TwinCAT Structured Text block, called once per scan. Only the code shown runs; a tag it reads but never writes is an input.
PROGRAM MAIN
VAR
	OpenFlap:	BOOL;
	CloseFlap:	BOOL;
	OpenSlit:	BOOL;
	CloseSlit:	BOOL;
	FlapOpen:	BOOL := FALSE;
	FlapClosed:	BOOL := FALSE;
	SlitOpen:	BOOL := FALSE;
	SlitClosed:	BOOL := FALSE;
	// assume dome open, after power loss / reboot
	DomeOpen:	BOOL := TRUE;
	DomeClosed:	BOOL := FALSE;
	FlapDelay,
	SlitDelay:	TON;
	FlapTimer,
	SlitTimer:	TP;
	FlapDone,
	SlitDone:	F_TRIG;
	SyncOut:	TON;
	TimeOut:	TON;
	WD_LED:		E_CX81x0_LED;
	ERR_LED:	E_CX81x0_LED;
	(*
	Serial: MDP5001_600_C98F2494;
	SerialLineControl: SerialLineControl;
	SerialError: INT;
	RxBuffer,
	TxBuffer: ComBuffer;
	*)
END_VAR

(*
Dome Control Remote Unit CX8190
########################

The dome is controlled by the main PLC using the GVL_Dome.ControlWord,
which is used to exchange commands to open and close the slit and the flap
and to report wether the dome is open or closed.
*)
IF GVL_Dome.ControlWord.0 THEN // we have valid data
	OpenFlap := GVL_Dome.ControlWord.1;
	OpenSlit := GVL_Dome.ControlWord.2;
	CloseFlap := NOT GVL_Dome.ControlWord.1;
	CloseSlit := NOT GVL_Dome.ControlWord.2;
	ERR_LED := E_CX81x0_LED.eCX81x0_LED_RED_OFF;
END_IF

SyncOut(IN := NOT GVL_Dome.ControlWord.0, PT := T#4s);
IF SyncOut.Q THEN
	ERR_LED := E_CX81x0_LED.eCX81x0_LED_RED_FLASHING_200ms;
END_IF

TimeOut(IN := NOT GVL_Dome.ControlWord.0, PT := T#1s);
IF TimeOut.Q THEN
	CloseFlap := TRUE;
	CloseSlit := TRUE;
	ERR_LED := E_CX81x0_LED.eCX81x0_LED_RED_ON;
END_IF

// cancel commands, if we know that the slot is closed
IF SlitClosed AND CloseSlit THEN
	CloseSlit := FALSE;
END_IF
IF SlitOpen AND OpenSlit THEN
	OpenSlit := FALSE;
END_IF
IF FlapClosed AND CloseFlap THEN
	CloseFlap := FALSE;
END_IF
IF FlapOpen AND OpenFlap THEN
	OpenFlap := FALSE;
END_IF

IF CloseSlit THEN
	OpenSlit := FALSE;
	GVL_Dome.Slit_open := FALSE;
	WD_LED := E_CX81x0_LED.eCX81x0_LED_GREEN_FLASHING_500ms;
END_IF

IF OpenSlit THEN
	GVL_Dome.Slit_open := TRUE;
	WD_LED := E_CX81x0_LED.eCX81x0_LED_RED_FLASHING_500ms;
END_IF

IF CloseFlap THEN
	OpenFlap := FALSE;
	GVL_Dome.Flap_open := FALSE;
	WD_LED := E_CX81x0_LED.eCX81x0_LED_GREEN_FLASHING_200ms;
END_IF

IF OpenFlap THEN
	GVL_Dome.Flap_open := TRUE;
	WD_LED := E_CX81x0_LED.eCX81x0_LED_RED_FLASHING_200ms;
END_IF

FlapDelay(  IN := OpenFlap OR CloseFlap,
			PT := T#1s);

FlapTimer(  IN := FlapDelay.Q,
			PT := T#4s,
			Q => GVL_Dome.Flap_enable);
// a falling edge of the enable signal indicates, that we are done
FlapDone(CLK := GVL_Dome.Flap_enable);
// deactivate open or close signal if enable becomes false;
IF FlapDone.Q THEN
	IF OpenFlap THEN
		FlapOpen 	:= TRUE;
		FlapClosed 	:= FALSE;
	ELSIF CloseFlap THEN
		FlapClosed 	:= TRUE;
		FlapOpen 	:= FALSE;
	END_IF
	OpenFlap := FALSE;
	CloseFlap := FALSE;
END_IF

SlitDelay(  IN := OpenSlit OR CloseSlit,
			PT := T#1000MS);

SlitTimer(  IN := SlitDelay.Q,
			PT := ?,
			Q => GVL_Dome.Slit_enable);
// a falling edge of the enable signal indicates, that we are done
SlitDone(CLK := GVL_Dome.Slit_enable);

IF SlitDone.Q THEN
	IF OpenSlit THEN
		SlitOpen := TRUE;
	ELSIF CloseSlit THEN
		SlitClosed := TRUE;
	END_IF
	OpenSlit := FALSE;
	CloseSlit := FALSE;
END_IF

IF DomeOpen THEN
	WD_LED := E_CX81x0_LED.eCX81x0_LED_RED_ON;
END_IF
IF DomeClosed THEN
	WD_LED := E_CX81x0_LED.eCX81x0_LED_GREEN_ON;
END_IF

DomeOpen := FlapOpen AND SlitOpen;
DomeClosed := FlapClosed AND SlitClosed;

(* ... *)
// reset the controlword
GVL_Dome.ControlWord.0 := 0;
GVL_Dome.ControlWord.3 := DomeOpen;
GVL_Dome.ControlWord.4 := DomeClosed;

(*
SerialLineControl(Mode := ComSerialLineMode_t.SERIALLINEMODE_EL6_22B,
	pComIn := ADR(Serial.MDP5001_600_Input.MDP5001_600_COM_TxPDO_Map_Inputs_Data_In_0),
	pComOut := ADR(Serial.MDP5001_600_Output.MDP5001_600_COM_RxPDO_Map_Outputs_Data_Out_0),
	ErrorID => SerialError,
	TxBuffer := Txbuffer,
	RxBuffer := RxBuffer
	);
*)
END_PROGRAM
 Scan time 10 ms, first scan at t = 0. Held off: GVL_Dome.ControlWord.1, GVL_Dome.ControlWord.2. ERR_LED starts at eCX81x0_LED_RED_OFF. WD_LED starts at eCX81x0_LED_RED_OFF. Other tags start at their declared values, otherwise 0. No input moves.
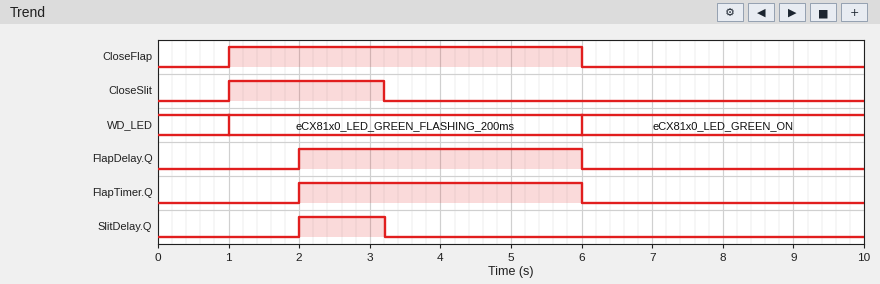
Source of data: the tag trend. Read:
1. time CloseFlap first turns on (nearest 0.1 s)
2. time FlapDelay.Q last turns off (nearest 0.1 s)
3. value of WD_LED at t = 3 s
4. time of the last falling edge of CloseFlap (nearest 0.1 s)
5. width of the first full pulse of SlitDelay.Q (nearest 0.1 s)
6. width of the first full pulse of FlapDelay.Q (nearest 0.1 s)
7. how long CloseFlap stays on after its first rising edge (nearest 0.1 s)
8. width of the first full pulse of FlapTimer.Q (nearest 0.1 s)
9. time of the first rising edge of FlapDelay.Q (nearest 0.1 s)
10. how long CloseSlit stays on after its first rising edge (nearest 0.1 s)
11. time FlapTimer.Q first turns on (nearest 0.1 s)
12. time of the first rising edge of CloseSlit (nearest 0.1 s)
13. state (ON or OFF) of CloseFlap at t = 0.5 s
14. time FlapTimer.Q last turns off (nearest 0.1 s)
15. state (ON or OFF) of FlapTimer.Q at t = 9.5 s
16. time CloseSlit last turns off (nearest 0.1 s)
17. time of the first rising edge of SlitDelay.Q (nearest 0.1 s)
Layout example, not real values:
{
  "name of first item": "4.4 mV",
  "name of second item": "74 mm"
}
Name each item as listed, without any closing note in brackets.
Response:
{
  "time CloseFlap first turns on": "1.0 s",
  "time FlapDelay.Q last turns off": "6.0 s",
  "value of WD_LED at t = 3 s": "eCX81x0_LED_GREEN_FLASHING_200ms",
  "time of the last falling edge of CloseFlap": "6.0 s",
  "width of the first full pulse of SlitDelay.Q": "1.2 s",
  "width of the first full pulse of FlapDelay.Q": "4.0 s",
  "how long CloseFlap stays on after its first rising edge": "5.0 s",
  "width of the first full pulse of FlapTimer.Q": "4.0 s",
  "time of the first rising edge of FlapDelay.Q": "2.0 s",
  "how long CloseSlit stays on after its first rising edge": "2.2 s",
  "time FlapTimer.Q first turns on": "2.0 s",
  "time of the first rising edge of CloseSlit": "1.0 s",
  "state (ON or OFF) of CloseFlap at t = 0.5 s": "OFF",
  "time FlapTimer.Q last turns off": "6.0 s",
  "state (ON or OFF) of FlapTimer.Q at t = 9.5 s": "OFF",
  "time CloseSlit last turns off": "3.2 s",
  "time of the first rising edge of SlitDelay.Q": "2.0 s"
}
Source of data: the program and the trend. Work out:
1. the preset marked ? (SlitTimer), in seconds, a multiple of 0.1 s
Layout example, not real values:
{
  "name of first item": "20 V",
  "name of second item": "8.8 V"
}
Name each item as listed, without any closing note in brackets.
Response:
{
  "the preset marked ? (SlitTimer), in seconds, a multiple of 0.1 s": "1.2 s"
}
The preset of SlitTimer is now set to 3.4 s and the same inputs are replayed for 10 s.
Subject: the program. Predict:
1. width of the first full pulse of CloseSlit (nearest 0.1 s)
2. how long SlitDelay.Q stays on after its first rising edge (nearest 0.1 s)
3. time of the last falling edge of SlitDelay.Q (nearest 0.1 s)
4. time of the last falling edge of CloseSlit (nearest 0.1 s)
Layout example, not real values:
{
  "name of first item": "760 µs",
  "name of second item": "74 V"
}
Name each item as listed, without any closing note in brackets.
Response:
{
  "width of the first full pulse of CloseSlit": "4.4 s",
  "how long SlitDelay.Q stays on after its first rising edge": "3.4 s",
  "time of the last falling edge of SlitDelay.Q": "5.4 s",
  "time of the last falling edge of CloseSlit": "5.4 s"
}
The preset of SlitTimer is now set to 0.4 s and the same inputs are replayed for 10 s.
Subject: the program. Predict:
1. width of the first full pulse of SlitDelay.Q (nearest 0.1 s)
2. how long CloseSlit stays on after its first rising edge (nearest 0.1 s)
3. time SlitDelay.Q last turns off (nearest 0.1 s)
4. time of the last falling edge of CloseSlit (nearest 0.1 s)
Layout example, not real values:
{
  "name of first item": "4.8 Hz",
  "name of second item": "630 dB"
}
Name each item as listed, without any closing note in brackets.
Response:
{
  "width of the first full pulse of SlitDelay.Q": "0.4 s",
  "how long CloseSlit stays on after its first rising edge": "1.4 s",
  "time SlitDelay.Q last turns off": "2.4 s",
  "time of the last falling edge of CloseSlit": "2.4 s"
}
